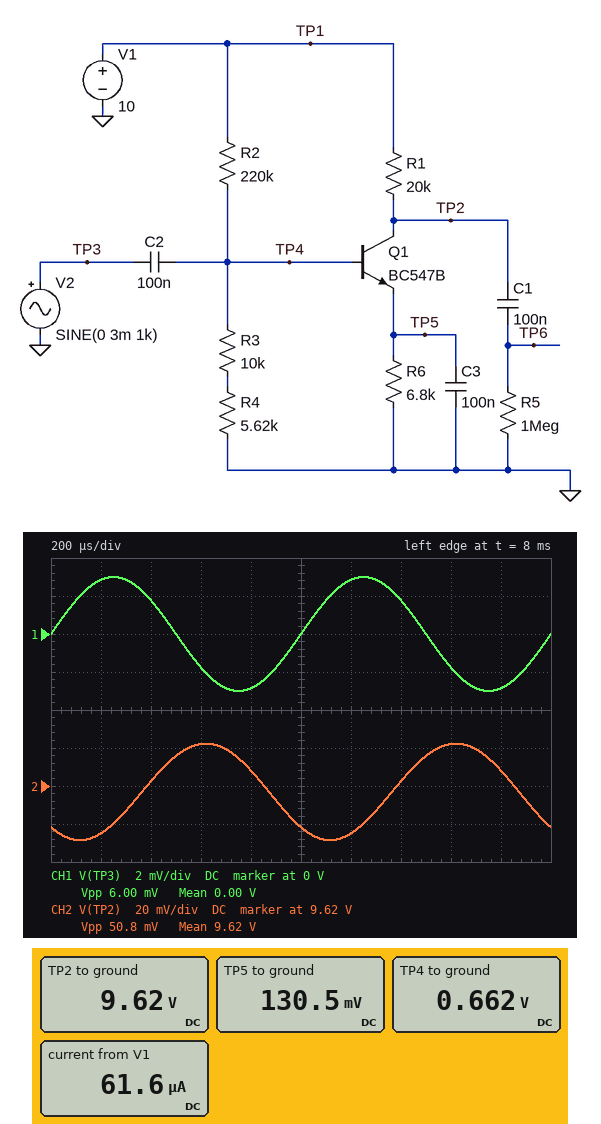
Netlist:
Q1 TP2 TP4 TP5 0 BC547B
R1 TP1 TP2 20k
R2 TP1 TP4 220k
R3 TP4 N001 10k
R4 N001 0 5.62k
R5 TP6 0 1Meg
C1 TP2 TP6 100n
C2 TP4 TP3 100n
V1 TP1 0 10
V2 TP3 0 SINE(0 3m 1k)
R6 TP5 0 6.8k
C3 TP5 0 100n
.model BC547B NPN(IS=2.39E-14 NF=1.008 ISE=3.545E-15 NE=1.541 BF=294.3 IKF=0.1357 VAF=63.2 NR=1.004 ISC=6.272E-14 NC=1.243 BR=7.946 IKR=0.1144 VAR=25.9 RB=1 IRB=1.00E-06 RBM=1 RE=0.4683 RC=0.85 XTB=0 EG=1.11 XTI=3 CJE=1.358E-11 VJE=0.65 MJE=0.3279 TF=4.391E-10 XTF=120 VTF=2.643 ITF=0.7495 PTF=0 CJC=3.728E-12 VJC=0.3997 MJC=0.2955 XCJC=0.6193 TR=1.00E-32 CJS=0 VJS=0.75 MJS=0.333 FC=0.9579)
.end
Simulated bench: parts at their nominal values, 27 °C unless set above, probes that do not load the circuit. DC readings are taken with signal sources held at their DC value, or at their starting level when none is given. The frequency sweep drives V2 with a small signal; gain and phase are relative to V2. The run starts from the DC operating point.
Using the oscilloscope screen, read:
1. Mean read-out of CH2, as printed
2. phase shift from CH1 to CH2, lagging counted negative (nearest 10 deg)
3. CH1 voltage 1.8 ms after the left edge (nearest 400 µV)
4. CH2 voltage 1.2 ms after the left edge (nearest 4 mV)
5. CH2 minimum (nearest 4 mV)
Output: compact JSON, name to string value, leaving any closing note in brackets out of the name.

{"Mean read-out of CH2, as printed": "9.62 V", "phase shift from CH1 to CH2, lagging counted negative": "-130 deg", "CH1 voltage 1.8 ms after the left edge": "-2.8 mV", "CH2 voltage 1.2 ms after the left edge": "9.596 V", "CH2 minimum": "9.592 V"}
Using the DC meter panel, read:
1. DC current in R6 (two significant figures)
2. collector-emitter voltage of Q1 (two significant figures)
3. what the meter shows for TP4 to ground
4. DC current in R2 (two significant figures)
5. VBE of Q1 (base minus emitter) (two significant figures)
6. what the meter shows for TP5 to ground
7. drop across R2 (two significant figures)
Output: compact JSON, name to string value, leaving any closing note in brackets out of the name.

{"DC current in R6": "19 µA", "collector-emitter voltage of Q1": "9.5 V", "what the meter shows for TP4 to ground": "0.662 V", "DC current in R2": "42 µA", "VBE of Q1 (base minus emitter)": "530 mV", "what the meter shows for TP5 to ground": "130.5 mV", "drop across R2": "9.3 V"}
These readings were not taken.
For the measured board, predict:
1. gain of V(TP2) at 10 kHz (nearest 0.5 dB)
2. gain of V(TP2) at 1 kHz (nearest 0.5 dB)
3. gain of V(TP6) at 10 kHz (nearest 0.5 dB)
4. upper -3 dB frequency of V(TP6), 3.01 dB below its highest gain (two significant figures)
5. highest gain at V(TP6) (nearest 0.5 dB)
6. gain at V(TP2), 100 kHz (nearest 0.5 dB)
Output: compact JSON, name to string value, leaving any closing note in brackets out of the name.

{"gain of V(TP2) at 10 kHz": "23.0 dB", "gain of V(TP2) at 1 kHz": "18.5 dB", "gain of V(TP6) at 10 kHz": "23.0 dB", "upper -3 dB frequency of V(TP6), 3.01 dB below its highest gain": "5.6 MHz", "highest gain at V(TP6)": "23.0 dB", "gain at V(TP2), 100 kHz": "23.0 dB"}
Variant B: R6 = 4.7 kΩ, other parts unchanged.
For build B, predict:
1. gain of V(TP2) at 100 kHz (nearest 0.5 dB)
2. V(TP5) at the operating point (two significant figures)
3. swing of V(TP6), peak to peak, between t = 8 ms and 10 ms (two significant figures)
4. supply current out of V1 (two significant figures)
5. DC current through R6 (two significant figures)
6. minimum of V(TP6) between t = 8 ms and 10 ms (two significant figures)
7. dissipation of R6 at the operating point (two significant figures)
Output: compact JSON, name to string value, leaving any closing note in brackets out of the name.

{"gain of V(TP2) at 100 kHz": "25.5 dB", "V(TP5) at the operating point": "120 mV", "swing of V(TP6), peak to peak, between t = 8 ms and 10 ms": "56 mV", "supply current out of V1": "68 µA", "DC current through R6": "26 µA", "minimum of V(TP6) between t = 8 ms and 10 ms": "-28 mV", "dissipation of R6 at the operating point": "3.2 µW"}
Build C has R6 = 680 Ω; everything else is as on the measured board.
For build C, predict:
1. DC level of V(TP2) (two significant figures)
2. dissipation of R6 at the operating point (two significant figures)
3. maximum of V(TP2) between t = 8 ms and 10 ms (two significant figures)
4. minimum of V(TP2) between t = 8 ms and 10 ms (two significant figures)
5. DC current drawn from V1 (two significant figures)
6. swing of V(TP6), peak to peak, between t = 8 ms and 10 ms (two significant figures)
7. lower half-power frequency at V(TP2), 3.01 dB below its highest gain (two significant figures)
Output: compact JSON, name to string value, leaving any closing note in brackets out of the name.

{"DC level of V(TP2)": "7.7 V", "dissipation of R6 at the operating point": "9.1 µW", "maximum of V(TP2) between t = 8 ms and 10 ms": "7.8 V", "minimum of V(TP2) between t = 8 ms and 10 ms": "7.6 V", "DC current drawn from V1": "160 µA", "swing of V(TP6), peak to peak, between t = 8 ms and 10 ms": "140 mV", "lower half-power frequency at V(TP2), 3.01 dB below its highest gain": "8.5 kHz"}
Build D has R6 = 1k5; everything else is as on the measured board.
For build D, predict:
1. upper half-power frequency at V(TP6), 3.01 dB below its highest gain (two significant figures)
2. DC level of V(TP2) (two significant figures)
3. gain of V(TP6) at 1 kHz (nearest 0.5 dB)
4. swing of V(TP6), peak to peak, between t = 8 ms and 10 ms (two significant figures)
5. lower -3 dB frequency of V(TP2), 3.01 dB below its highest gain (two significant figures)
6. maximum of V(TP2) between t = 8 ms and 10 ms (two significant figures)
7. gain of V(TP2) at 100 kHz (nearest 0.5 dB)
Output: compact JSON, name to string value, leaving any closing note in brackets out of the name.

{"upper half-power frequency at V(TP6), 3.01 dB below its highest gain": "5.5 MHz", "DC level of V(TP2)": "8.7 V", "gain of V(TP6) at 1 kHz": "22.5 dB", "swing of V(TP6), peak to peak, between t = 8 ms and 10 ms": "82 mV", "lower -3 dB frequency of V(TP2), 3.01 dB below its highest gain": "4.7 kHz", "maximum of V(TP2) between t = 8 ms and 10 ms": "8.8 V", "gain of V(TP2) at 100 kHz": "33.5 dB"}
